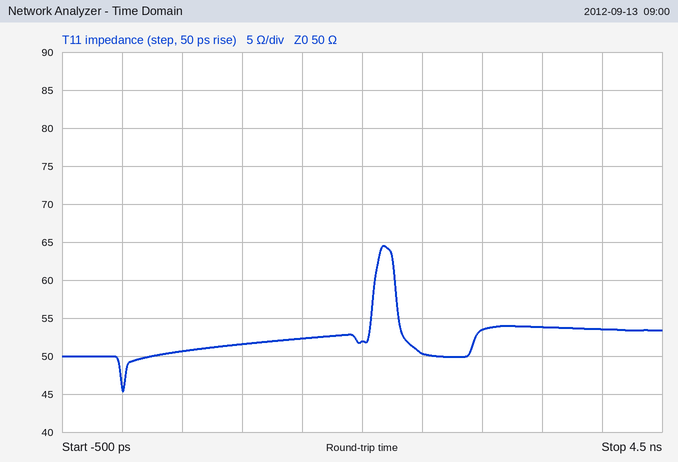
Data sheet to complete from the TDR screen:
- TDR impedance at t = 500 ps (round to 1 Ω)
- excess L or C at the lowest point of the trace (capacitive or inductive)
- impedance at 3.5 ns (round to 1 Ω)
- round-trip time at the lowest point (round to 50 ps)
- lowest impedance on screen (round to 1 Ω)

51 Ω
capacitive
54 Ω
0 ps
45 Ω
